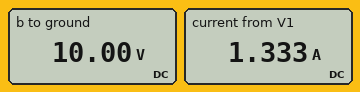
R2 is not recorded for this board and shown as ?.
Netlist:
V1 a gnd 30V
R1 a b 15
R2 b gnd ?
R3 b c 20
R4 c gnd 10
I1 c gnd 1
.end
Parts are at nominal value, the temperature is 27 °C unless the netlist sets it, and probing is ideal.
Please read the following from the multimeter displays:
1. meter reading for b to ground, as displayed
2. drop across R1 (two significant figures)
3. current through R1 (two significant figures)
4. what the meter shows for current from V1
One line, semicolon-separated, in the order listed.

10.00 V; 20 V; 1.3 A; 1.333 A
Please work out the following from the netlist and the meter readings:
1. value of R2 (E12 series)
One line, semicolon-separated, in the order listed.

15 Ω
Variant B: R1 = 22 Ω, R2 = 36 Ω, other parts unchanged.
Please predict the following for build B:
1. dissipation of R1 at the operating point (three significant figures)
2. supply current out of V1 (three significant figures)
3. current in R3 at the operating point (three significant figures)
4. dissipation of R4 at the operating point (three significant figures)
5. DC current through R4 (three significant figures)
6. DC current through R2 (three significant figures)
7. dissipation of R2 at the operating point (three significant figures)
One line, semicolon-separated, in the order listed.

18.8 W; 924 mA; 656 mA; 1.19 W; 344 mA; 269 mA; 2.60 W
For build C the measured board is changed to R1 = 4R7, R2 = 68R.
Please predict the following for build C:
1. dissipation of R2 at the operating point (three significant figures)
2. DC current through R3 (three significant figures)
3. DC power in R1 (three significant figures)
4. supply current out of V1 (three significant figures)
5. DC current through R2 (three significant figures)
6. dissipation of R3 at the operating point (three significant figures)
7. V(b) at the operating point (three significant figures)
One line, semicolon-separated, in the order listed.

7.91 W; 1.11 A; 9.85 W; 1.45 A; 341 mA; 24.5 W; 23.2 V
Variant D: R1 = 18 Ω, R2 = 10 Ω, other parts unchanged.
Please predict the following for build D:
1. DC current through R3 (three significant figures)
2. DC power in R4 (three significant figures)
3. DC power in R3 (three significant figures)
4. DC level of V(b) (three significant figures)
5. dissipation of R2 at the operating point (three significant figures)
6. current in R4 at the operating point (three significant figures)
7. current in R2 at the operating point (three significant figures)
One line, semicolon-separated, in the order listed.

569 mA; 1.86 W; 6.47 W; 7.06 V; 4.98 W; 431 mA; 706 mA
